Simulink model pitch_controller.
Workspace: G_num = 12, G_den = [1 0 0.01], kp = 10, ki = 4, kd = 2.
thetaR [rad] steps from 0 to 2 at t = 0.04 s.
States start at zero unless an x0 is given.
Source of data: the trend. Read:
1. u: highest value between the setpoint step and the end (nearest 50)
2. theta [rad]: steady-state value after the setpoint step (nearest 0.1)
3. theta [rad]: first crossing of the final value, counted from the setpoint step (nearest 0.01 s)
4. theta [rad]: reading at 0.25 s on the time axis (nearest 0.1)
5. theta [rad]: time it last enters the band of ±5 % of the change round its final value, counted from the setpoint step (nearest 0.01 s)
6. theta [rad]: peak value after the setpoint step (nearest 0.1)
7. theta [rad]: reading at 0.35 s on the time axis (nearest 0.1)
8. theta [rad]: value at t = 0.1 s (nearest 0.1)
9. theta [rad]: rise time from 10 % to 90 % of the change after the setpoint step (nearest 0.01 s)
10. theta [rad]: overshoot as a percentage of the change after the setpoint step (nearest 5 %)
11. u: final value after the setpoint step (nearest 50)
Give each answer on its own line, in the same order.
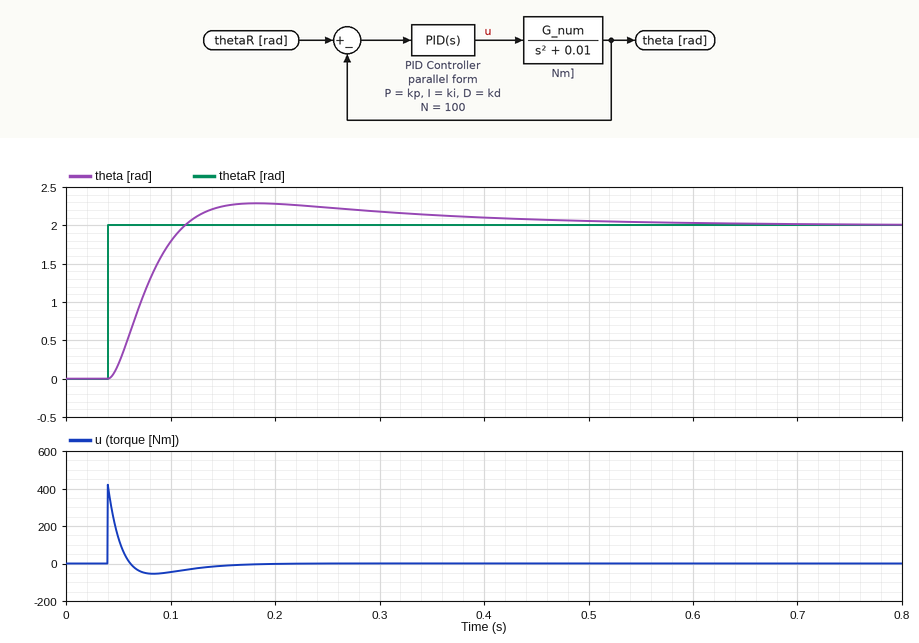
400
2.0
0.07 s
2.2
0.36 s
2.3
2.1
1.8
0.05 s
15 %
0
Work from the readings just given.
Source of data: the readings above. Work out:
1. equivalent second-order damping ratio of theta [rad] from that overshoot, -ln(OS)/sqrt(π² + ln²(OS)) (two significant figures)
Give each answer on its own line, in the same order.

0.52
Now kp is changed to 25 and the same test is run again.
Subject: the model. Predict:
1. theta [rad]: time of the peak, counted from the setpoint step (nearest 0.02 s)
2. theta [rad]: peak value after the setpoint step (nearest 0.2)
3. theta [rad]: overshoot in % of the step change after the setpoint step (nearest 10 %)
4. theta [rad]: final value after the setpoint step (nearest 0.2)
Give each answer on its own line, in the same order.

0.10 s
2.6
30 %
2.0
